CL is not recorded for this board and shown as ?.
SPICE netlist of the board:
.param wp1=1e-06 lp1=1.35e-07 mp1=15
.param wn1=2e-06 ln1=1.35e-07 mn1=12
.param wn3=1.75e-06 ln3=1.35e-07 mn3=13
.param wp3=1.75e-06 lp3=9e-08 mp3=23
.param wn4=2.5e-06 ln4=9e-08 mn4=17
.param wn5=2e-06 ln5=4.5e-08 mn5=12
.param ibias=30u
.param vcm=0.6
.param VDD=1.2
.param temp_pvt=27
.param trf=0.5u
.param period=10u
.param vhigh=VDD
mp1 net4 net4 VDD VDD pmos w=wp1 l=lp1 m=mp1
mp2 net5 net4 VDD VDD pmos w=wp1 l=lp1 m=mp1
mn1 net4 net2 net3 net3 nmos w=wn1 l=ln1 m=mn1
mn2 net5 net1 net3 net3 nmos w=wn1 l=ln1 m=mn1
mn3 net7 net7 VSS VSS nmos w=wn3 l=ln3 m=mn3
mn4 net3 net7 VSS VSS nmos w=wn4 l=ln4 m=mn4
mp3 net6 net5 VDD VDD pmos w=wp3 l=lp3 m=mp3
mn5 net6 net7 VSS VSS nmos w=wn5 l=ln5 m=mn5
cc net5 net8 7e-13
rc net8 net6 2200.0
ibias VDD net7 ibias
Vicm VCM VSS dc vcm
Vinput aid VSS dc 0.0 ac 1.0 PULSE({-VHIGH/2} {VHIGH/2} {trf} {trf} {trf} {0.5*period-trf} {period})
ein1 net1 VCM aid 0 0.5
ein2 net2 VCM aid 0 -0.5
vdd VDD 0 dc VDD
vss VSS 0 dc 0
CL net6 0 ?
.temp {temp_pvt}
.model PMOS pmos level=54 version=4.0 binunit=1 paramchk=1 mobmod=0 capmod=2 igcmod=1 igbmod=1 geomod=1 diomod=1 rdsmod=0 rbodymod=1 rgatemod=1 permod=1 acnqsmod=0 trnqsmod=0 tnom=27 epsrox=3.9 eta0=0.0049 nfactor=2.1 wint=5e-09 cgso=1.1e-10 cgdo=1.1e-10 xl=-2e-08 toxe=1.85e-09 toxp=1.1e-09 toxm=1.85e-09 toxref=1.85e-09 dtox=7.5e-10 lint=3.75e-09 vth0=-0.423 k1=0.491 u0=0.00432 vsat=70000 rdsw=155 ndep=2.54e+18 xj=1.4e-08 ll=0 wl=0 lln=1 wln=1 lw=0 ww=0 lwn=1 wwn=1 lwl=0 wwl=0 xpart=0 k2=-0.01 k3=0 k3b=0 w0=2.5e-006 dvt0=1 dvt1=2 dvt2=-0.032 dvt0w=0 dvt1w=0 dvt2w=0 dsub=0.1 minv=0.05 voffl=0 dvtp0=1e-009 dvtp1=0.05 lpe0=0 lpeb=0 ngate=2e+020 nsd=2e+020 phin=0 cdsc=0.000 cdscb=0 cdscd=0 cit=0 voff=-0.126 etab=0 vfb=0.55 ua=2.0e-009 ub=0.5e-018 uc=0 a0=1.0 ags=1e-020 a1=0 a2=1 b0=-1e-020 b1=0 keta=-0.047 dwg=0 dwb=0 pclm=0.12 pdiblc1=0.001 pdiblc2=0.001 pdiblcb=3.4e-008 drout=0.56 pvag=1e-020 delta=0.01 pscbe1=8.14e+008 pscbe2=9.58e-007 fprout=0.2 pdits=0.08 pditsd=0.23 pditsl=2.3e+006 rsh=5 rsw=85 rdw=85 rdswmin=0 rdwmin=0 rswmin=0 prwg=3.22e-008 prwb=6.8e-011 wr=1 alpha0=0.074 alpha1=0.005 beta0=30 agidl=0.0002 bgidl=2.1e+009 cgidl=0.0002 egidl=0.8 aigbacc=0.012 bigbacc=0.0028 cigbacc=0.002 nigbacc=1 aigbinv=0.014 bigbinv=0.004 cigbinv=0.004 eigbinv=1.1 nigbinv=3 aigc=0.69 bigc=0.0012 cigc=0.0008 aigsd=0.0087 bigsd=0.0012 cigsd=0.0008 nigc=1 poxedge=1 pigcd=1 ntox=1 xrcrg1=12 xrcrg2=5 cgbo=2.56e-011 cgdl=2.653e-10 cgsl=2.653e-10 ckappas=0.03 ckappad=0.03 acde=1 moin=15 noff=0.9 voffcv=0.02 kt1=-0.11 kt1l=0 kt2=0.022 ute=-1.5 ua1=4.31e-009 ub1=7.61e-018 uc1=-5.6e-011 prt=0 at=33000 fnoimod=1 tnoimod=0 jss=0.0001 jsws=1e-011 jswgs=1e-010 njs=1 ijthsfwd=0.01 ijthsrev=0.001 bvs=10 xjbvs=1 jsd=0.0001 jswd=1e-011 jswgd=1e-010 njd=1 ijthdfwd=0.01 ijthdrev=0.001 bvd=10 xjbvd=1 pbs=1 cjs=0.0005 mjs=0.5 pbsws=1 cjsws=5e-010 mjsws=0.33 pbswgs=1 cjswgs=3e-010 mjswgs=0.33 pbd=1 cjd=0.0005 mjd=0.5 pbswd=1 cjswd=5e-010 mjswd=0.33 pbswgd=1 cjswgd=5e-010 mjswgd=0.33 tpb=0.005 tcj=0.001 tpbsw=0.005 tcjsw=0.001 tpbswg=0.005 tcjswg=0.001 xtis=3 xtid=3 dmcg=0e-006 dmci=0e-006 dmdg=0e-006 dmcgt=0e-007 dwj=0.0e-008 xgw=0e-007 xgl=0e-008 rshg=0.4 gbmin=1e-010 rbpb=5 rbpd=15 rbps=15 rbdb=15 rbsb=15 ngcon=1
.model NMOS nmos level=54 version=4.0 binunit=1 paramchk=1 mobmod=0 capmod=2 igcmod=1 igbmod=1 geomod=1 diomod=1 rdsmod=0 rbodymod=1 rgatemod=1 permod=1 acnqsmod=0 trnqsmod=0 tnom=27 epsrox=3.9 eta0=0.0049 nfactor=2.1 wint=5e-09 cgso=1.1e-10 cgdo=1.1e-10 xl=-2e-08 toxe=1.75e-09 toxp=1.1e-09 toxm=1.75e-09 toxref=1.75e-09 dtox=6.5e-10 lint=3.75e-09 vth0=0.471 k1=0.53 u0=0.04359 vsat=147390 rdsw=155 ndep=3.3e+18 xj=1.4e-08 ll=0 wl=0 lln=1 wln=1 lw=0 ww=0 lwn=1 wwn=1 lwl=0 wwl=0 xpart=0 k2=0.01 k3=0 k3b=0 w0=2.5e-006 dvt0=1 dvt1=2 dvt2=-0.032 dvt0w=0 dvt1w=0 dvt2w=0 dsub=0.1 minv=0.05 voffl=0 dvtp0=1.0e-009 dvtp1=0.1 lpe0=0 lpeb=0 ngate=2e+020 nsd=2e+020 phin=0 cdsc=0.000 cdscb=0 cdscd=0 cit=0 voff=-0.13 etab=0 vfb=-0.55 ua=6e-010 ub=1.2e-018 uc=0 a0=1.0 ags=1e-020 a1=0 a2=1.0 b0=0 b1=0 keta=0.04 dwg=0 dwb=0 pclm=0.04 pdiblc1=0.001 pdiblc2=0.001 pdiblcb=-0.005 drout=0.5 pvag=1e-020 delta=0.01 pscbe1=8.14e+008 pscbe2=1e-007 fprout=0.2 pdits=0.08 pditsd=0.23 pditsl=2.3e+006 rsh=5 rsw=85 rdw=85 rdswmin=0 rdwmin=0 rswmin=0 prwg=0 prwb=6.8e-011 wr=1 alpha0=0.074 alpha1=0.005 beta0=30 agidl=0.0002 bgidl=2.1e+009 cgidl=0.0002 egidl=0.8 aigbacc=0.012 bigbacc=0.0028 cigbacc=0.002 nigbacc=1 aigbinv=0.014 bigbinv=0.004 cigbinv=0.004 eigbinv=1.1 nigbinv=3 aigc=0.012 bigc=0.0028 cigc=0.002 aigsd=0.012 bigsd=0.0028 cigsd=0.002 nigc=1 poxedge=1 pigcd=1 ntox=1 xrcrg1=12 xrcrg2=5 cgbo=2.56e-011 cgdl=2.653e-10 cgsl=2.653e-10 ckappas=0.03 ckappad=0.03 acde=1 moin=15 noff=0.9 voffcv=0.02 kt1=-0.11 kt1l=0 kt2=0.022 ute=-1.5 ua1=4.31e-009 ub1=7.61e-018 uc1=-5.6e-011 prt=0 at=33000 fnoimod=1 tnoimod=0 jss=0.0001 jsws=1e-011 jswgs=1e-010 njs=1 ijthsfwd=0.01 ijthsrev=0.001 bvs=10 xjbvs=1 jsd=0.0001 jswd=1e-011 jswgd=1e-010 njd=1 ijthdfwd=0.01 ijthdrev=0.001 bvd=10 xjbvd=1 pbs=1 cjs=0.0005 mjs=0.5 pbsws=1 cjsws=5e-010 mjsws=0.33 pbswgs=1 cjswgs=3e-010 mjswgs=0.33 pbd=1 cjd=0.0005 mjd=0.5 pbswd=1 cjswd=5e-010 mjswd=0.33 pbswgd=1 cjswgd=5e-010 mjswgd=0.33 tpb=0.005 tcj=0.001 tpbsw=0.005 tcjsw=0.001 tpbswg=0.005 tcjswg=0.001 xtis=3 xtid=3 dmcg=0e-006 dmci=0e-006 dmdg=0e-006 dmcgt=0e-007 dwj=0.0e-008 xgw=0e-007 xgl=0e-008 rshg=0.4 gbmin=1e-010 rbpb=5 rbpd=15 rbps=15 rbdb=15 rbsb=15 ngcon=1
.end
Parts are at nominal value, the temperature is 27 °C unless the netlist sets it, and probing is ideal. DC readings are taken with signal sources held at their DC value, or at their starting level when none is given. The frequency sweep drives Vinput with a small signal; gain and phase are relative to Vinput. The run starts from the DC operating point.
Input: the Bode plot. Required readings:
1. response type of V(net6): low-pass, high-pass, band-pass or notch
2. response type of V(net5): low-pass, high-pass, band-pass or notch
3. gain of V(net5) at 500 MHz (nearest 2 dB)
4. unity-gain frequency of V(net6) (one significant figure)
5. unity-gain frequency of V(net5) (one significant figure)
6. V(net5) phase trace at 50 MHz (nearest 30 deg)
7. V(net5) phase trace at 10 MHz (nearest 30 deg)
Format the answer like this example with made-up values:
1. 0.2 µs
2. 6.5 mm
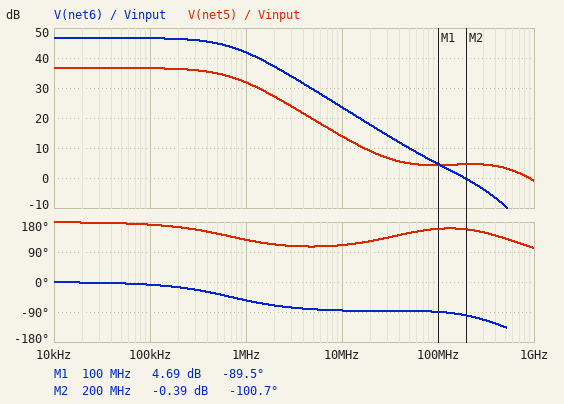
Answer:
1. low-pass
2. low-pass
3. 4 dB
4. 200 MHz
5. 900 MHz
6. 150 deg
7. 120 deg
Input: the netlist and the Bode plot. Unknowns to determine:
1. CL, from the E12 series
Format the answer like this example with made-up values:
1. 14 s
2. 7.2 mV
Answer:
1. 3.9 pF
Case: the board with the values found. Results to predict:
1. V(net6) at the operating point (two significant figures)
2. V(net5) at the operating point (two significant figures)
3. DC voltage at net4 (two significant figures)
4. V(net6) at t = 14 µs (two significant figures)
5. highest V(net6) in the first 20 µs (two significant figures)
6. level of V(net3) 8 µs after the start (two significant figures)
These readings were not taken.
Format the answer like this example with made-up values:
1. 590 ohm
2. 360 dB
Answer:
1. 140 mV
2. 670 mV
3. 670 mV
4. 1.0 V
5. 1.0 V
6. 460 mV
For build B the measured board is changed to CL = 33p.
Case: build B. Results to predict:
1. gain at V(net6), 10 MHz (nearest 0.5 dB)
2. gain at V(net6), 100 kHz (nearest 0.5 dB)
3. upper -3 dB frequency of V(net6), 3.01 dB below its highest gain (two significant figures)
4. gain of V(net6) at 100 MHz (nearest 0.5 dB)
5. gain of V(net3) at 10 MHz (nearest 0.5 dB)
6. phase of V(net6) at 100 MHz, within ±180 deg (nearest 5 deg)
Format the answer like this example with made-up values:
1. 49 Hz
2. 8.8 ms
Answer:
1. 22.0 dB
2. 46.5 dB
3. 640 kHz
4. -8.5 dB
5. -27.0 dB
6. -140 deg
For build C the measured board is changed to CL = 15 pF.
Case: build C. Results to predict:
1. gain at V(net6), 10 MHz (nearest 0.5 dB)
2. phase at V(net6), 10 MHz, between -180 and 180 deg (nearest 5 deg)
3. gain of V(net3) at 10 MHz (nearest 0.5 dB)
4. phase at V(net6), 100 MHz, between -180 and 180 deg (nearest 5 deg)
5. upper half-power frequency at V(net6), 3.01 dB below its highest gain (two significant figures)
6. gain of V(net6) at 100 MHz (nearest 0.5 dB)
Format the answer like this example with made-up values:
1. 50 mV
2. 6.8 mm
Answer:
1. 23.0 dB
2. -95 deg
3. -29.0 dB
4. -125 deg
5. 680 kHz
6. -2.0 dB
